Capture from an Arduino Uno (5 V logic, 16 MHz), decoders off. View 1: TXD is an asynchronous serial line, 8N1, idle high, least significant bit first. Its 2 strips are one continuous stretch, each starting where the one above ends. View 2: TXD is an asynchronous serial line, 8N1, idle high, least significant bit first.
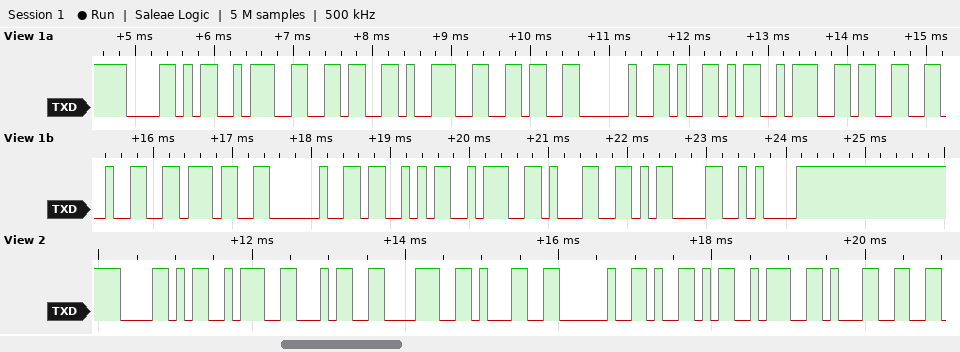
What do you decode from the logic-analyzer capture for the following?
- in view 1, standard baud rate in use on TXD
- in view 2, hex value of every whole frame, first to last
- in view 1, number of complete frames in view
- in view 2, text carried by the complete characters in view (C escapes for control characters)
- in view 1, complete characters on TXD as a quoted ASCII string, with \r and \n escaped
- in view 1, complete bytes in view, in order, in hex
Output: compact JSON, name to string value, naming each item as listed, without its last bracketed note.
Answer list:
{"in view 1, standard baud rate in use on TXD": "9600 baud", "in view 2, hex value of every whole frame, first to last": "58 3A 34 38 31 20 59 3A 31", "in view 1, number of complete frames in view": "17", "in view 2, text carried by the complete characters in view": "\"X:481 Y:1\"", "in view 1, complete characters on TXD as a quoted ASCII string, with \\r and \\n escaped": "\"X:696 Y:327 S:1\\r\\n\"", "in view 1, complete bytes in view, in order, in hex": "58 3A 36 39 36 20 59 3A 33 32 37 20 53 3A 31 0D 0A"}
